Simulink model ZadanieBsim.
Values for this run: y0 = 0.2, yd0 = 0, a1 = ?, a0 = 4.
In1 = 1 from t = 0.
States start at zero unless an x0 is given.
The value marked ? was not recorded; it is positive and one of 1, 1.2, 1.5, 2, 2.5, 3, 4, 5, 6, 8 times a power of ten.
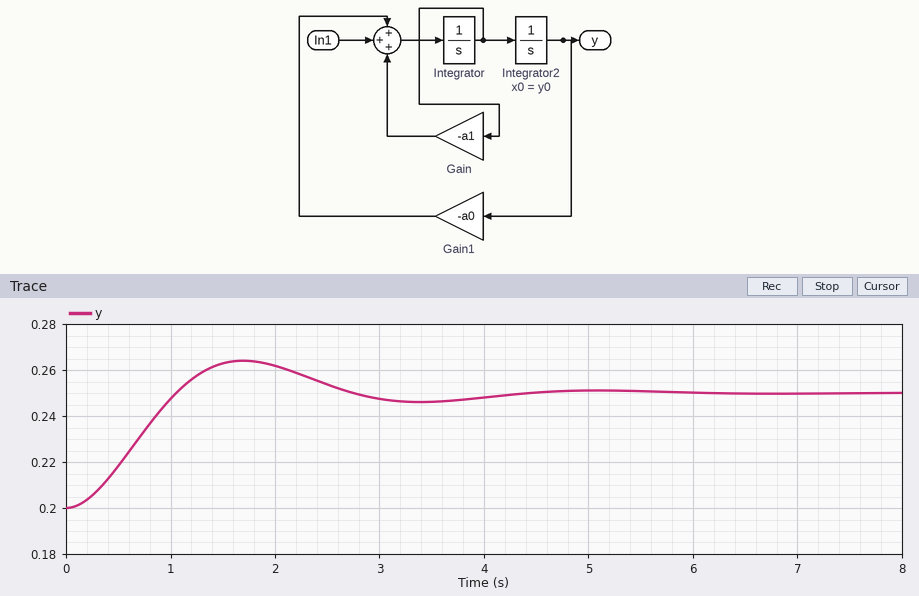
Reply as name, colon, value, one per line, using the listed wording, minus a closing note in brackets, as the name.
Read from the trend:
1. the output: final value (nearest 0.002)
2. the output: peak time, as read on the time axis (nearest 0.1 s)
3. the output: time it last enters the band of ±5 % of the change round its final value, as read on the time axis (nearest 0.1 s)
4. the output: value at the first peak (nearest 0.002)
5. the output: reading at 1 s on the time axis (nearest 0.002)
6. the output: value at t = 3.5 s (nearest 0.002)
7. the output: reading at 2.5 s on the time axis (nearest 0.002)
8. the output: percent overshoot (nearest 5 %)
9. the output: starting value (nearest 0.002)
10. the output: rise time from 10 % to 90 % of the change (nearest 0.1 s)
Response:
the output: final value: 0.250
the output: peak time, as read on the time axis: 1.7 s
the output: time it last enters the band of ±5 % of the change round its final value, as read on the time axis: 3.9 s
the output: value at the first peak: 0.264
the output: reading at 1 s on the time axis: 0.248
the output: value at t = 3.5 s: 0.246
the output: reading at 2.5 s on the time axis: 0.254
the output: percent overshoot: 30 %
the output: starting value: 0.200
the output: rise time from 10 % to 90 % of the change: 0.7 s
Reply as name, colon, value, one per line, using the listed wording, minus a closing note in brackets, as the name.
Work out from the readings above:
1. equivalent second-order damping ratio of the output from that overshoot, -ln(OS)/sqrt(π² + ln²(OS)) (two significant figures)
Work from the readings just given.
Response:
equivalent second-order damping ratio of the output from that overshoot, -ln(OS)/sqrt(π² + ln²(OS)): 0.36
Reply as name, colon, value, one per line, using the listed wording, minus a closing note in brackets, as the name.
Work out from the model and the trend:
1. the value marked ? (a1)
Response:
the value marked ?: 1.5
